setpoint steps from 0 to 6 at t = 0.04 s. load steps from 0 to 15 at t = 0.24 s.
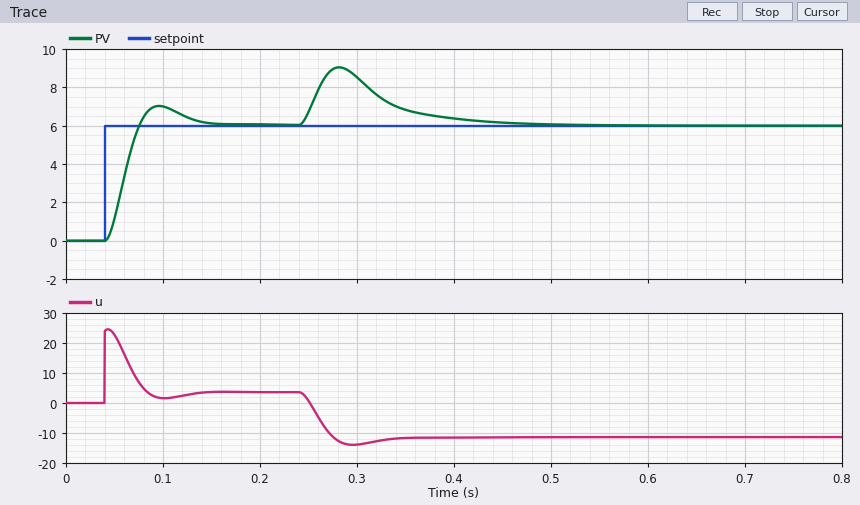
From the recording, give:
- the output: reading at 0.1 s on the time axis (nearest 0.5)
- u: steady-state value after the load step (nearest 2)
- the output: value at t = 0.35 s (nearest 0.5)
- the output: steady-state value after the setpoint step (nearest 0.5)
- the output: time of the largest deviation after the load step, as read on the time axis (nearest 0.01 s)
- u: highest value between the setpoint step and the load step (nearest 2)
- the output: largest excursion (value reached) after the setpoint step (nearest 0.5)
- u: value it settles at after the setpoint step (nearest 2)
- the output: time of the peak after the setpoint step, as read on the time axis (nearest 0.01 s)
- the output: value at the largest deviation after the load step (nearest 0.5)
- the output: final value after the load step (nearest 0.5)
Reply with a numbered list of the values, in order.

1. 7.0
2. -12
3. 7.0
4. 6.0
5. 0.28 s
6. 24
7. 7.0
8. 4
9. 0.10 s
10. 9.0
11. 6.0
